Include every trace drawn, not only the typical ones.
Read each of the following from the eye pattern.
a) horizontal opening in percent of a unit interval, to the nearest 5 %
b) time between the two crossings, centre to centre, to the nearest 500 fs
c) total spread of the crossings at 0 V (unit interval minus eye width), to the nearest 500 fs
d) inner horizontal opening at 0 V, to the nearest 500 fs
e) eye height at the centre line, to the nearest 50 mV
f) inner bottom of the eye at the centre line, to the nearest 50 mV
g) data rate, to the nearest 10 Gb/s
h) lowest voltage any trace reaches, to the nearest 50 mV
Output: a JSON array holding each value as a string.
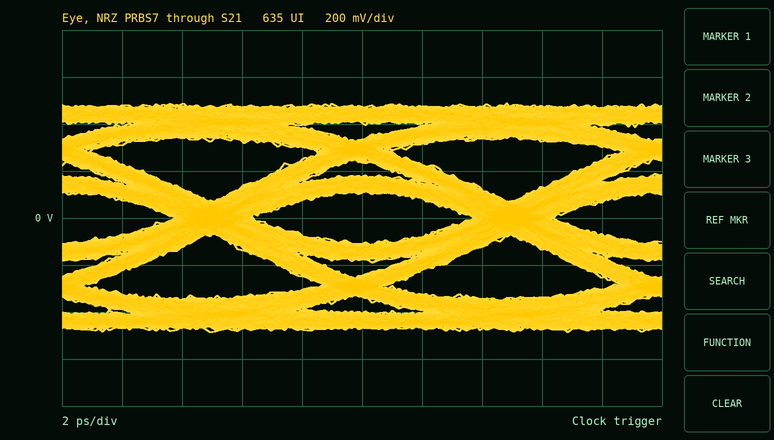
["75 %", "10.0 ps", "2.5 ps", "7.5 ps", "200 mV", "-100 mV", "100 Gb/s", "-500 mV"]
